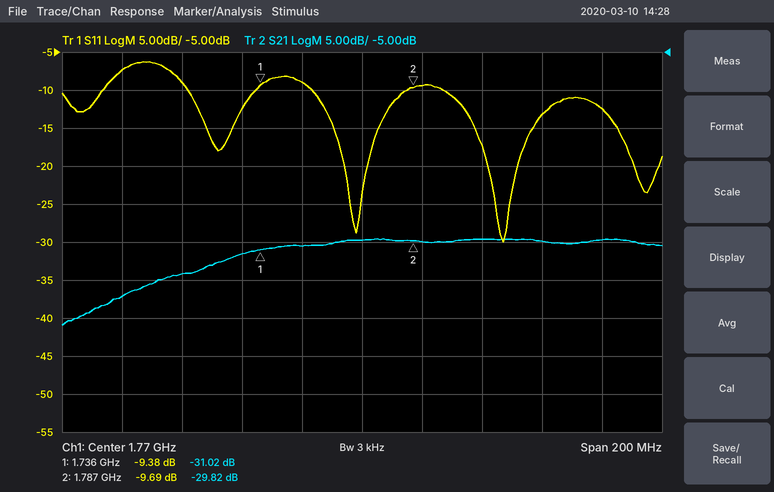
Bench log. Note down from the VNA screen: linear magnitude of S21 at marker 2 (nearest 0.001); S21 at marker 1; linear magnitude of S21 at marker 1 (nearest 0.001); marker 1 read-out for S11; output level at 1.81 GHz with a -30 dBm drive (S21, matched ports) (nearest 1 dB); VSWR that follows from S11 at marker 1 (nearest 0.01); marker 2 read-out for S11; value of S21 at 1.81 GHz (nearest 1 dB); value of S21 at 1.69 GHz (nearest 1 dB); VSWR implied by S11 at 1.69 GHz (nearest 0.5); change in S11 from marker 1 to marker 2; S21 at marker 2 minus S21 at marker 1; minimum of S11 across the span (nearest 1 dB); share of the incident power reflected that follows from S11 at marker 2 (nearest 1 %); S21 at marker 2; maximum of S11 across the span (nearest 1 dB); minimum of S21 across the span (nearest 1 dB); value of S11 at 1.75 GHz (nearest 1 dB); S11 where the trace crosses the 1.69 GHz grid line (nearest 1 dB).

0.032
-31.02 dB
0.028
-9.38 dB
-60 dBm
2.03
-9.69 dB
-30 dB
-37 dB
2.5
-0.31 dB
1.20 dB
-30 dB
11 %
-29.82 dB
-6 dB
-41 dB
-9 dB
-7 dB
